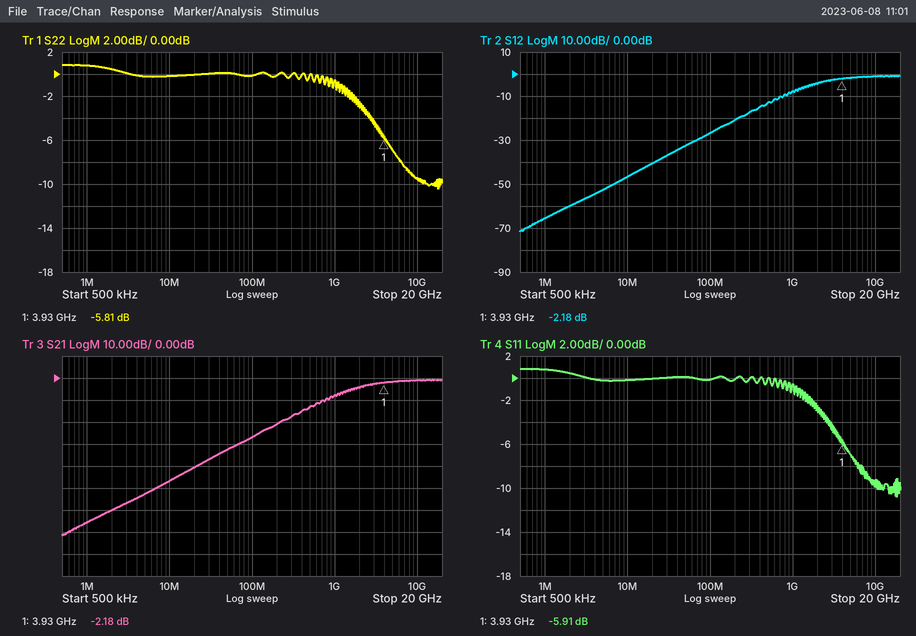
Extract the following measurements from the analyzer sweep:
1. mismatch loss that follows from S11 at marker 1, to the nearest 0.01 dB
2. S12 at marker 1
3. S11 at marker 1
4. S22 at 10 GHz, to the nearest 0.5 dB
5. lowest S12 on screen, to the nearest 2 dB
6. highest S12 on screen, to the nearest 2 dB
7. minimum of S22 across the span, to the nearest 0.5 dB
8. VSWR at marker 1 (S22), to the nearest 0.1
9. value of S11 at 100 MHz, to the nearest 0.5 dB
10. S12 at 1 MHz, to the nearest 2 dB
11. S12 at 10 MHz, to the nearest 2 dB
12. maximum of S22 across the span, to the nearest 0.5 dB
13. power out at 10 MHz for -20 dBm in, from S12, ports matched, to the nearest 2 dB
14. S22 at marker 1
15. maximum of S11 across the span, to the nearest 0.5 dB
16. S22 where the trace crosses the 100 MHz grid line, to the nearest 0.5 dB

1.29 dB
-2.18 dB
-5.91 dB
-9.5 dB
-72 dB
0 dB
-10.5 dB
3.1
0.0 dB
-66 dB
-46 dB
1.0 dB
-66 dBm
-5.81 dB
1.0 dB
0.0 dB
